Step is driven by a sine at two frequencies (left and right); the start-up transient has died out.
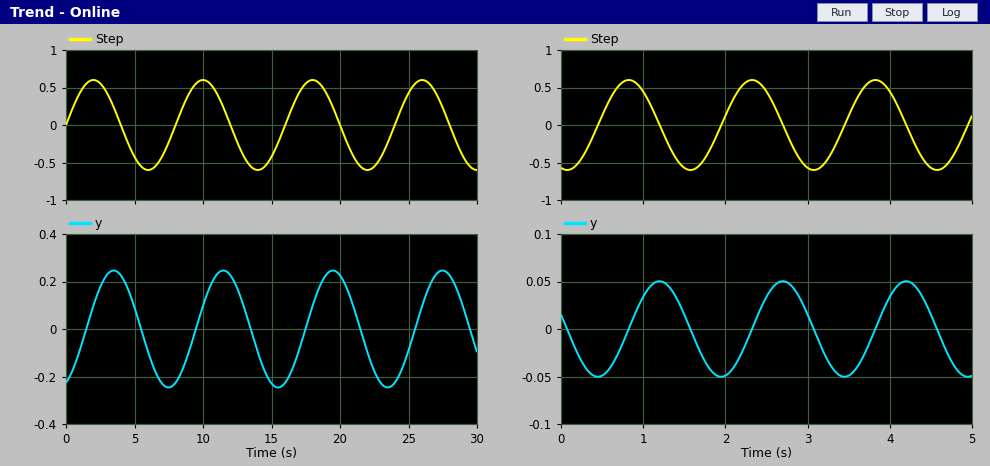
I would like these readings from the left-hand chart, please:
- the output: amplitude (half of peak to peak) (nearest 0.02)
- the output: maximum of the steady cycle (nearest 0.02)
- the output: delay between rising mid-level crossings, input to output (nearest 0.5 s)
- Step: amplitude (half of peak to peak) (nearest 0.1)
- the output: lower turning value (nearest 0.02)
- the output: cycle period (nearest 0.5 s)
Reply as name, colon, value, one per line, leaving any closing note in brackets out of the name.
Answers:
the output: amplitude (half of peak to peak): 0.24
the output: maximum of the steady cycle: 0.24
the output: delay between rising mid-level crossings, input to output: 1.5 s
Step: amplitude (half of peak to peak): 0.6
the output: lower turning value: -0.24
the output: cycle period: 8.0 s
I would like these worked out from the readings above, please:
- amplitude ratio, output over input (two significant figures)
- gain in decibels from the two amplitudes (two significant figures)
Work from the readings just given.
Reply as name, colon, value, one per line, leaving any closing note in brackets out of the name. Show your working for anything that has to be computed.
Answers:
amplitude ratio, output over input: 0.24 / 0.6 = 0.40
gain in decibels from the two amplitudes: 20 log10(0.24 / 0.6) = -8.0 dB
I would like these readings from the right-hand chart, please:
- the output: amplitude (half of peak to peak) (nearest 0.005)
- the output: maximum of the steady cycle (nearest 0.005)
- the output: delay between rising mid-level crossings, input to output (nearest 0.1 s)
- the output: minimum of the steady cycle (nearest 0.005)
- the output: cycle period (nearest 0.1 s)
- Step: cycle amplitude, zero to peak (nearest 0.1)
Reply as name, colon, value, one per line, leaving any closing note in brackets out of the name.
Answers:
the output: amplitude (half of peak to peak): 0.050
the output: maximum of the steady cycle: 0.050
the output: delay between rising mid-level crossings, input to output: 0.4 s
the output: minimum of the steady cycle: -0.050
the output: cycle period: 1.5 s
Step: cycle amplitude, zero to peak: 0.6
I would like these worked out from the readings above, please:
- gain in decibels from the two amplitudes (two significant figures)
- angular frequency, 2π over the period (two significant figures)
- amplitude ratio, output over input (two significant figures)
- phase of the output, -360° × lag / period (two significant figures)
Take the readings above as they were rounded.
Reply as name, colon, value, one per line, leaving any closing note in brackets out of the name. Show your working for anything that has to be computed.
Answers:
gain in decibels from the two amplitudes: 20 log10(0.05 / 0.6) = -22 dB
angular frequency, 2π over the period: 2π / 1.5 = 4.2 rad/s
amplitude ratio, output over input: 0.05 / 0.6 = 0.083
phase of the output, -360° × lag / period: -360 × 0.4 / 1.5 = -96°
